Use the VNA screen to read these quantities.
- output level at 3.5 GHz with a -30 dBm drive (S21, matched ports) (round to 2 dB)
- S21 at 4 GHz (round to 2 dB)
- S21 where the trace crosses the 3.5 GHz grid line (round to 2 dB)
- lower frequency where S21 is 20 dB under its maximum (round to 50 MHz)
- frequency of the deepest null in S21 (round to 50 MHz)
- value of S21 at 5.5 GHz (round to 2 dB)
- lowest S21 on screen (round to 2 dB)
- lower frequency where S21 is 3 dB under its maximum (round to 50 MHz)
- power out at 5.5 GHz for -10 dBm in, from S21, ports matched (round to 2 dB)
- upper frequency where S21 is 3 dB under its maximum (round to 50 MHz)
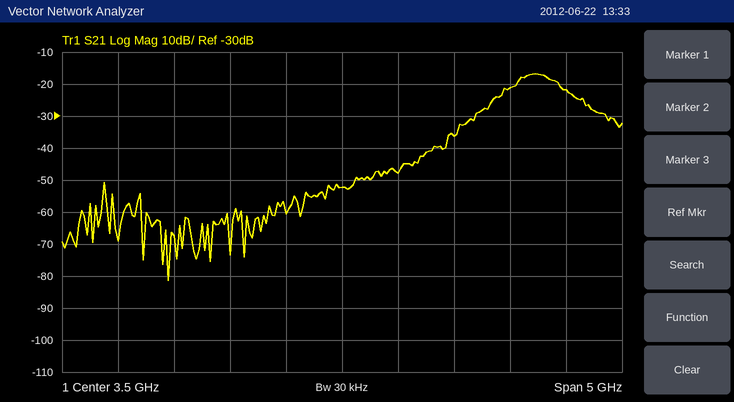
-82 dBm
-48 dB
-52 dB
4.45 GHz
1.95 GHz
-22 dB
-82 dB
5.05 GHz
-32 dBm
5.45 GHz
